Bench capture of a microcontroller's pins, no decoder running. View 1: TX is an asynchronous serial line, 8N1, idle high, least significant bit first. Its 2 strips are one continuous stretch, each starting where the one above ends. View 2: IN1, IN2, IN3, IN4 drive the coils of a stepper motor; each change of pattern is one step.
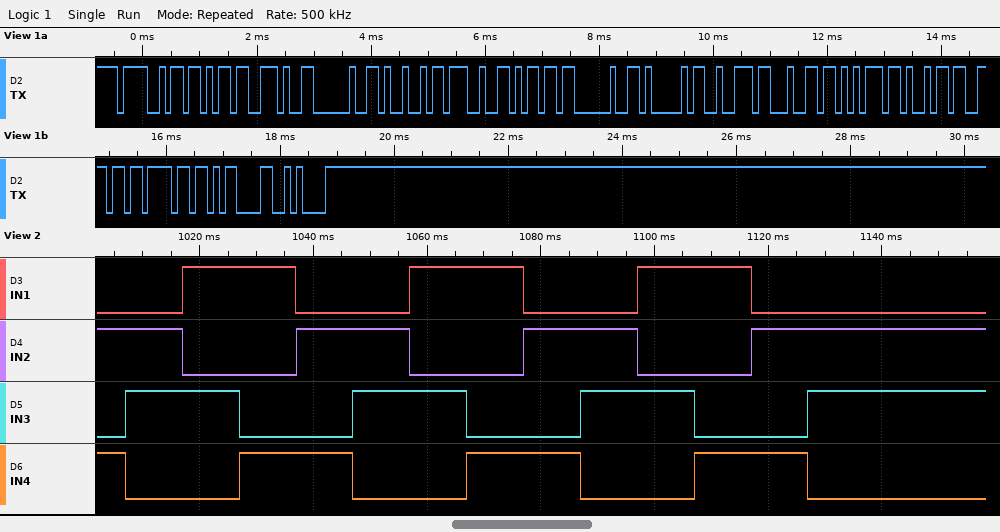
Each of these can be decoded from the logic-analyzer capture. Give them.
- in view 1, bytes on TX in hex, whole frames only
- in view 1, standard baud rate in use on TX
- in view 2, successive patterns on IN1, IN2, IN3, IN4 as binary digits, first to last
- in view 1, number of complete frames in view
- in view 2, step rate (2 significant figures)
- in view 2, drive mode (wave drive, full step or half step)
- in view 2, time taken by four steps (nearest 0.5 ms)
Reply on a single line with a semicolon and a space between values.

0x4F 0x6B 0x2E 0x20 0x49 0x27 0x6D 0x20 0x41 0x72 0x64 0x75 0x69 0x6E 0x6F 0x0D 0x0A; 9600 baud; 0101 0110 1010 1001 0101 0110 1010 1001 0101 0110 1010 1001 0101 0110; 17; 100 steps/s; full step; 40.0 ms
